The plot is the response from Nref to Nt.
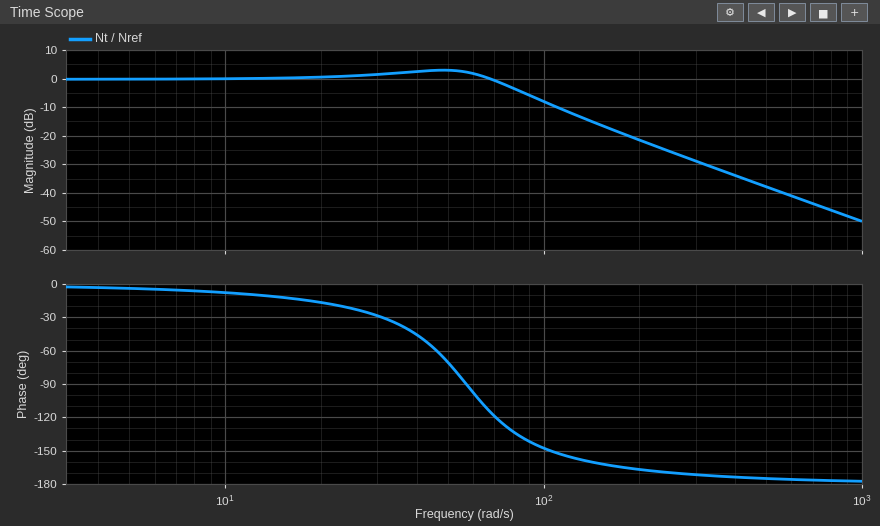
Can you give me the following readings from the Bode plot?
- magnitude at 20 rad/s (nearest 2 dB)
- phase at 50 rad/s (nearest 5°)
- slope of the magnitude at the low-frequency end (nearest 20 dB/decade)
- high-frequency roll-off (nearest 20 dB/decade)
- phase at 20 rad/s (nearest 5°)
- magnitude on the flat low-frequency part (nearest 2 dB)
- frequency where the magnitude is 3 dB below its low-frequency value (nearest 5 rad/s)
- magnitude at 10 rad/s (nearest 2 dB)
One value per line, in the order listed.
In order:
0 dB
-70°
0 dB/decade
-40 dB/decade
-15°
0 dB
80 rad/s
0 dB
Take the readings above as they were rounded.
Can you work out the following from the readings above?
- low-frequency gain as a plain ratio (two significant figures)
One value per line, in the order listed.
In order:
1.0
